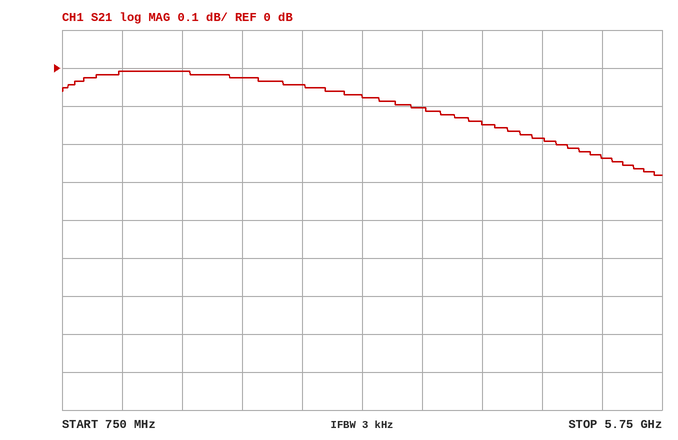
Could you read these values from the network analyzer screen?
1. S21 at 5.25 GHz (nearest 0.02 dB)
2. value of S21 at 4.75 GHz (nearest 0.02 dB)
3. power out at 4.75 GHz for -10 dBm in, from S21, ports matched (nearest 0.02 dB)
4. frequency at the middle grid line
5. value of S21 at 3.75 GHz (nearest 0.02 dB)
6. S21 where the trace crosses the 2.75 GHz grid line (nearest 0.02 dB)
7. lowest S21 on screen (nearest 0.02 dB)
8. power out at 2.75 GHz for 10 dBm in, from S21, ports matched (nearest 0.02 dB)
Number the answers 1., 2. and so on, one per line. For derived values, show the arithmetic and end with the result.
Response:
1. -0.24 dB
2. -0.18 dB
3. -10 dBm + (-0.18 dB) = -10.18 dBm
4. 3.25 GHz
5. -0.10 dB
6. -0.04 dB
7. -0.28 dB
8. 10 dBm + (-0.04 dB) = 9.96 dBm
